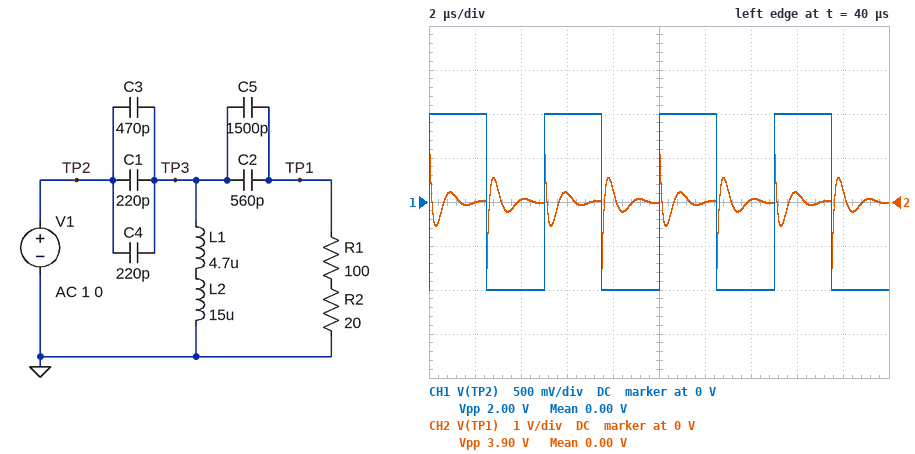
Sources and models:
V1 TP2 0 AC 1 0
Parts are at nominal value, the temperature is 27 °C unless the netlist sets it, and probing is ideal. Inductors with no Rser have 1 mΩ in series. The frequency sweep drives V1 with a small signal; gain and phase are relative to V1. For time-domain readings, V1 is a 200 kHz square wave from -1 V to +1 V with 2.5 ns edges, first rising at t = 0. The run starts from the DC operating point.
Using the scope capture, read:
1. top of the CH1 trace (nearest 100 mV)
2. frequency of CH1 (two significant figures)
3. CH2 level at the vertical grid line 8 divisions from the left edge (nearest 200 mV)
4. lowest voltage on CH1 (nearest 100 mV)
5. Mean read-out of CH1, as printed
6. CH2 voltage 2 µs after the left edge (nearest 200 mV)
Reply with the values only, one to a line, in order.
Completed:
1.0 V
200 kHz
200 mV
-1.0 V
0.00 V
0 V
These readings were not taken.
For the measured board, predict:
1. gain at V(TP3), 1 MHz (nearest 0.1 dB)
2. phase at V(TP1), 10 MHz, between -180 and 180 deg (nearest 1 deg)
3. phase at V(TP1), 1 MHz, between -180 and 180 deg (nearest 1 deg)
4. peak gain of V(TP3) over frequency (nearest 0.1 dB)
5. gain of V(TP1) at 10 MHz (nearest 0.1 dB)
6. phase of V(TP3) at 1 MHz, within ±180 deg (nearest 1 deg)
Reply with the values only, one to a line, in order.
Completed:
-0.5 dB
12 deg
109 deg
0 dB
-0.1 dB
76 deg
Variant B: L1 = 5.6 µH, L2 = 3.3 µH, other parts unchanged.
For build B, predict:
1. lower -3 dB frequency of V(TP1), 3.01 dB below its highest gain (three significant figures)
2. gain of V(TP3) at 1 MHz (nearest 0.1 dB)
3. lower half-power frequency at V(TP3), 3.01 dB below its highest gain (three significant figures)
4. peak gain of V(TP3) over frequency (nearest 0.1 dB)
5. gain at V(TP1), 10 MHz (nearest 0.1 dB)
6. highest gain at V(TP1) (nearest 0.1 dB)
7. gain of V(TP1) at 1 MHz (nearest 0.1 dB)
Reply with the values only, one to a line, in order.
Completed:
1.27 MHz
-5.1 dB
1.23 MHz
2.2 dB
0.1 dB
1.7 dB
-6.6 dB
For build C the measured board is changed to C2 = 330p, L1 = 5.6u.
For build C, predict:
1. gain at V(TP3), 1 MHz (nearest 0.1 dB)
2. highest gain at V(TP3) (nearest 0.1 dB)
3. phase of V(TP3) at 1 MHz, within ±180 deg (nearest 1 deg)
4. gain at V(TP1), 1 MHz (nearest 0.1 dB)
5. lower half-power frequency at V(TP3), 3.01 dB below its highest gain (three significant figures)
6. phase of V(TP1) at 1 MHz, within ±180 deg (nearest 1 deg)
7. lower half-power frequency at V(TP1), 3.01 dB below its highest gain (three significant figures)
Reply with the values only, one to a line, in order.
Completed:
-0.1 dB
0.1 dB
70 deg
-2.0 dB
663 kHz
106 deg
784 kHz
